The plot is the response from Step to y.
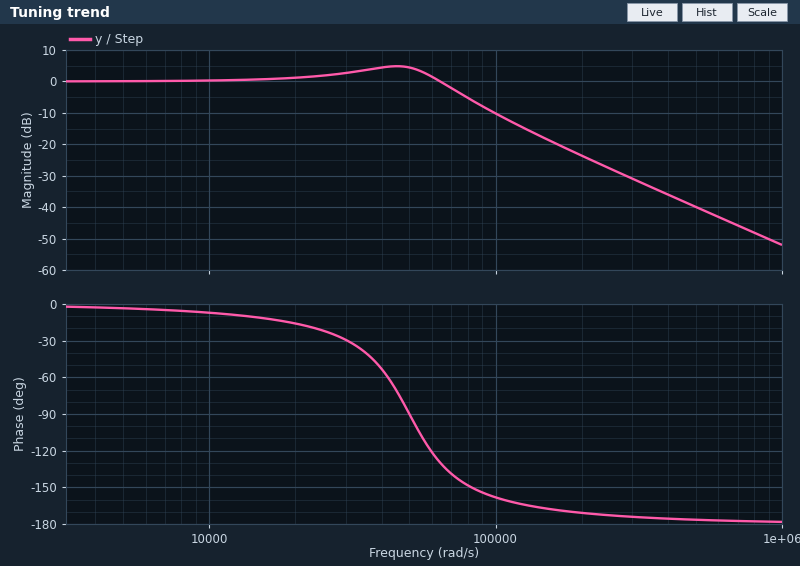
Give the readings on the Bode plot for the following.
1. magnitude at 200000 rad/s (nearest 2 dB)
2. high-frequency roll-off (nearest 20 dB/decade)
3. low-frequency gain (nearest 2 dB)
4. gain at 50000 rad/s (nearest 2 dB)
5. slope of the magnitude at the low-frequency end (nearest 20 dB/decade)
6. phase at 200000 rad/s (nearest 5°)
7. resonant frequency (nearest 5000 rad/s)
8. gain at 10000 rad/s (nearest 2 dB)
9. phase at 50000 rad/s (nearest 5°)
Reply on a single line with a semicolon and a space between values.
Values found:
-24 dB; -40 dB/decade; 0 dB; 4 dB; 0 dB/decade; -170°; 45000 rad/s; 0 dB; -90°
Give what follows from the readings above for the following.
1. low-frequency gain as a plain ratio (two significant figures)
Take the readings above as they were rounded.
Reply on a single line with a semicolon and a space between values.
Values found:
1.0
